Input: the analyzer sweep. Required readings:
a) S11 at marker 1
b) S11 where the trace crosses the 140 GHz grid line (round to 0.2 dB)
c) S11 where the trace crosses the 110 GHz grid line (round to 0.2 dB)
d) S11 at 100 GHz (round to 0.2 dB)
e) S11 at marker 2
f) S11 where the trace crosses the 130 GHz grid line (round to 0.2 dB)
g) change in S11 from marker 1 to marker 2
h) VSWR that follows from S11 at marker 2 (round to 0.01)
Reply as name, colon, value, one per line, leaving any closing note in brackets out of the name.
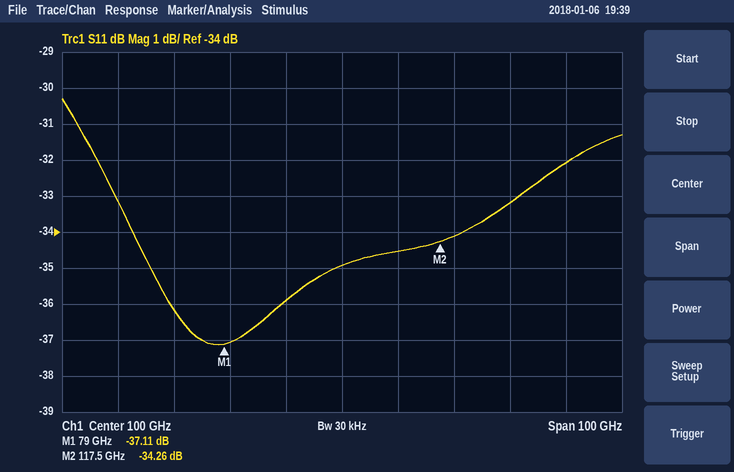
S11 at marker 1: -37.11 dB
S11 where the trace crosses the 140 GHz grid line: -32.0 dB
S11 where the trace crosses the 110 GHz grid line: -34.6 dB
S11 at 100 GHz: -35.0 dB
S11 at marker 2: -34.26 dB
S11 where the trace crosses the 130 GHz grid line: -33.2 dB
change in S11 from marker 1 to marker 2: 2.85 dB
VSWR that follows from S11 at marker 2: 1.04
